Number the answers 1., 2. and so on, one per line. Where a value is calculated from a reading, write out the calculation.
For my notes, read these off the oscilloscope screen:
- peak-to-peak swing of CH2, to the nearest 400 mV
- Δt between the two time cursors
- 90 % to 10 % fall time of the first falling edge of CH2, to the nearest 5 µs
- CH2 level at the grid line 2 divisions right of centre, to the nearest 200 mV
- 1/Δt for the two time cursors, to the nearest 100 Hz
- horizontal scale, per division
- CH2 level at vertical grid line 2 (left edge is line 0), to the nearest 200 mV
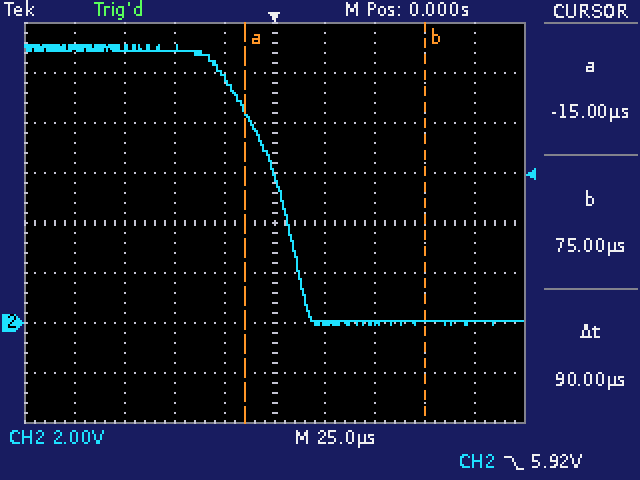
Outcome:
1. 11.2 V
2. 90 µs
3. 40 µs
4. 0.0 V
5. 1 / 90 µs ≈ 11.1 kHz
6. 25 µs
7. 11.0 V
